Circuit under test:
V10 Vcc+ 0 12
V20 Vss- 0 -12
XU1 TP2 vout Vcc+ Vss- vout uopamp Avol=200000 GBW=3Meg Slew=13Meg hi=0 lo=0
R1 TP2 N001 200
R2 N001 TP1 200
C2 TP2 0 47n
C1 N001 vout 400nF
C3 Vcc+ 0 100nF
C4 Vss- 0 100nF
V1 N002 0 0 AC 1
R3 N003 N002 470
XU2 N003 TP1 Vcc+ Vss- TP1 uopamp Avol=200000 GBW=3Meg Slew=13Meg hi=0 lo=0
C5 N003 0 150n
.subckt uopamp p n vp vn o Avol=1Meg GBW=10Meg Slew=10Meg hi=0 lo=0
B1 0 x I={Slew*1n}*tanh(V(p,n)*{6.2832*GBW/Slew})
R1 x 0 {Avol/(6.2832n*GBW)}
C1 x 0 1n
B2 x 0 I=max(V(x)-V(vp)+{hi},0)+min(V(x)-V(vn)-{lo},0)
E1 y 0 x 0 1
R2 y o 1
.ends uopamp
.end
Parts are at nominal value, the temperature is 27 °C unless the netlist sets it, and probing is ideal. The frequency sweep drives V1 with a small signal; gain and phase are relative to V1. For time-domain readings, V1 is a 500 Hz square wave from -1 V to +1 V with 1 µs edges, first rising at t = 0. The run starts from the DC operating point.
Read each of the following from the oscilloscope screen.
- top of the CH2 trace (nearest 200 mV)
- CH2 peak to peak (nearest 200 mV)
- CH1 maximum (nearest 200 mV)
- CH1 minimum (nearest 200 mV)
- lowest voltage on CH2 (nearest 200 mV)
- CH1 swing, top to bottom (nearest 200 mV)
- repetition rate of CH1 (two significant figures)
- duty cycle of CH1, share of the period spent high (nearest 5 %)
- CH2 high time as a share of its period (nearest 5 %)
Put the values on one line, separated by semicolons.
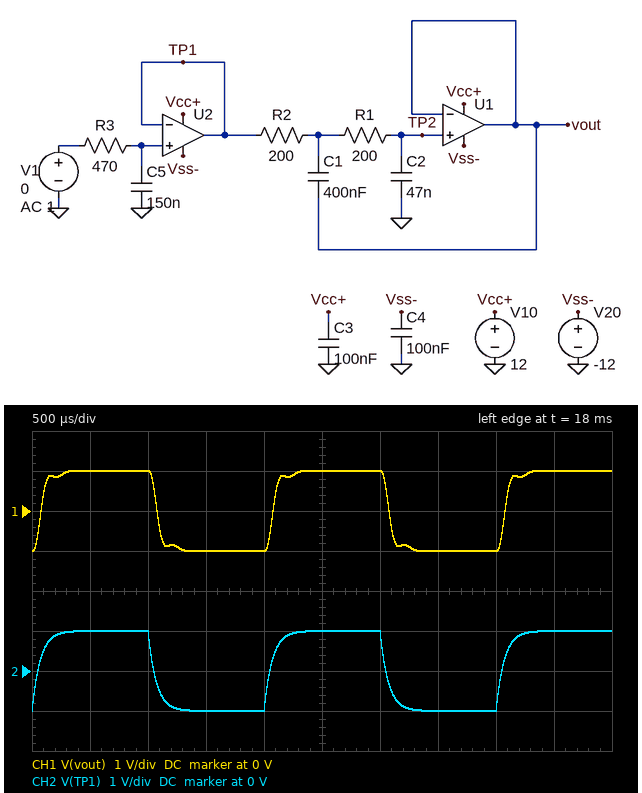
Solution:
1.0 V; 2.0 V; 1.0 V; -1.0 V; -1.0 V; 2.0 V; 500 Hz; 50 %; 50 %
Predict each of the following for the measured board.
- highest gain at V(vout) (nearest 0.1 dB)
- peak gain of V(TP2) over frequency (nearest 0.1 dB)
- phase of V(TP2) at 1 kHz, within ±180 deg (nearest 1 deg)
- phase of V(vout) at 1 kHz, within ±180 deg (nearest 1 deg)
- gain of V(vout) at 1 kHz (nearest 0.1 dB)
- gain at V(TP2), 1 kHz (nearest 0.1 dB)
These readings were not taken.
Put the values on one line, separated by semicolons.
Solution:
0 dB; 0 dB; -31 deg; -31 deg; -0.6 dB; -0.6 dB
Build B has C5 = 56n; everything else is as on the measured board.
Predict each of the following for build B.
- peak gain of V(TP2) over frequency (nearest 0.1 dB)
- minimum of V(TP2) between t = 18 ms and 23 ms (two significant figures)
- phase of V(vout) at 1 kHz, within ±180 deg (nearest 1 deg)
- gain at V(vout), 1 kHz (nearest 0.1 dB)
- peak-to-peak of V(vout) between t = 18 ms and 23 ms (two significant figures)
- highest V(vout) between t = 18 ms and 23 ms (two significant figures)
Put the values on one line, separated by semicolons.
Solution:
1.7 dB; -1.4 V; -16 deg; 0.1 dB; 2.8 V; 1.4 V
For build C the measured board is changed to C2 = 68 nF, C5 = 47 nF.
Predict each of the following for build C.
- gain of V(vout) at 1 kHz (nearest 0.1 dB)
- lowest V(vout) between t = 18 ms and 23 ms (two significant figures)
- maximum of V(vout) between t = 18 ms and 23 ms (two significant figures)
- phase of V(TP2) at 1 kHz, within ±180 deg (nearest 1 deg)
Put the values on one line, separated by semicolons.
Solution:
0.2 dB; -1.4 V; 1.4 V; -18 deg
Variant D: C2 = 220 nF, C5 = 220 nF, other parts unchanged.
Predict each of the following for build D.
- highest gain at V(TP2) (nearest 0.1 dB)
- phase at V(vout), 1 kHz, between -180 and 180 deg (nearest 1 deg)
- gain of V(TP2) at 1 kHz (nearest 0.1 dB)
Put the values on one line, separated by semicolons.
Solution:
0 dB; -66 deg; -1.7 dB
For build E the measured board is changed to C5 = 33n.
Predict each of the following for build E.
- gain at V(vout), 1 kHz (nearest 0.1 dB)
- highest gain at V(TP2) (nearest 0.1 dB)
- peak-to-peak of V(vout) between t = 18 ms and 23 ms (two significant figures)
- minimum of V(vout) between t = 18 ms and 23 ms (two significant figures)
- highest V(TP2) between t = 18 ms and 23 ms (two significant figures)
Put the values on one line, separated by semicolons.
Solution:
0.2 dB; 2.9 dB; 3.1 V; -1.5 V; 1.5 V
